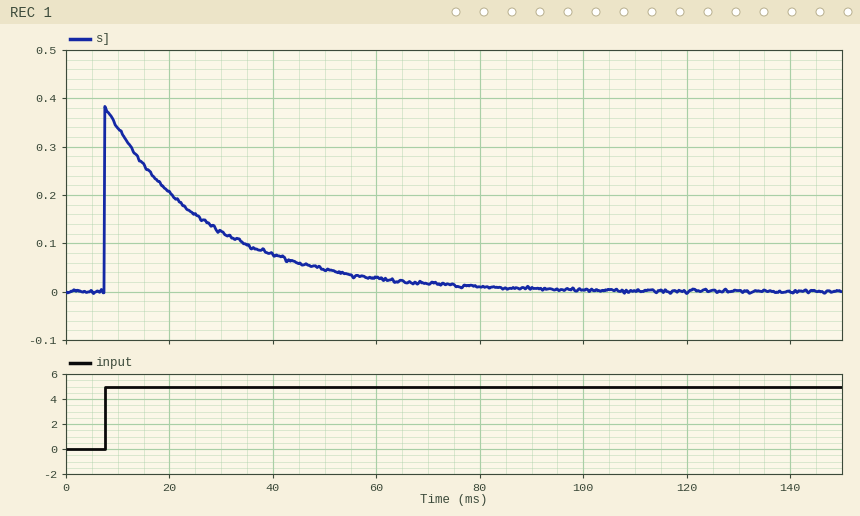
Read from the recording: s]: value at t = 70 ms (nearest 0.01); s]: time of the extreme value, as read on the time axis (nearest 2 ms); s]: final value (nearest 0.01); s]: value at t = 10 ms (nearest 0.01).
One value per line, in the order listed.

0.02
8 ms
0.00
0.34
